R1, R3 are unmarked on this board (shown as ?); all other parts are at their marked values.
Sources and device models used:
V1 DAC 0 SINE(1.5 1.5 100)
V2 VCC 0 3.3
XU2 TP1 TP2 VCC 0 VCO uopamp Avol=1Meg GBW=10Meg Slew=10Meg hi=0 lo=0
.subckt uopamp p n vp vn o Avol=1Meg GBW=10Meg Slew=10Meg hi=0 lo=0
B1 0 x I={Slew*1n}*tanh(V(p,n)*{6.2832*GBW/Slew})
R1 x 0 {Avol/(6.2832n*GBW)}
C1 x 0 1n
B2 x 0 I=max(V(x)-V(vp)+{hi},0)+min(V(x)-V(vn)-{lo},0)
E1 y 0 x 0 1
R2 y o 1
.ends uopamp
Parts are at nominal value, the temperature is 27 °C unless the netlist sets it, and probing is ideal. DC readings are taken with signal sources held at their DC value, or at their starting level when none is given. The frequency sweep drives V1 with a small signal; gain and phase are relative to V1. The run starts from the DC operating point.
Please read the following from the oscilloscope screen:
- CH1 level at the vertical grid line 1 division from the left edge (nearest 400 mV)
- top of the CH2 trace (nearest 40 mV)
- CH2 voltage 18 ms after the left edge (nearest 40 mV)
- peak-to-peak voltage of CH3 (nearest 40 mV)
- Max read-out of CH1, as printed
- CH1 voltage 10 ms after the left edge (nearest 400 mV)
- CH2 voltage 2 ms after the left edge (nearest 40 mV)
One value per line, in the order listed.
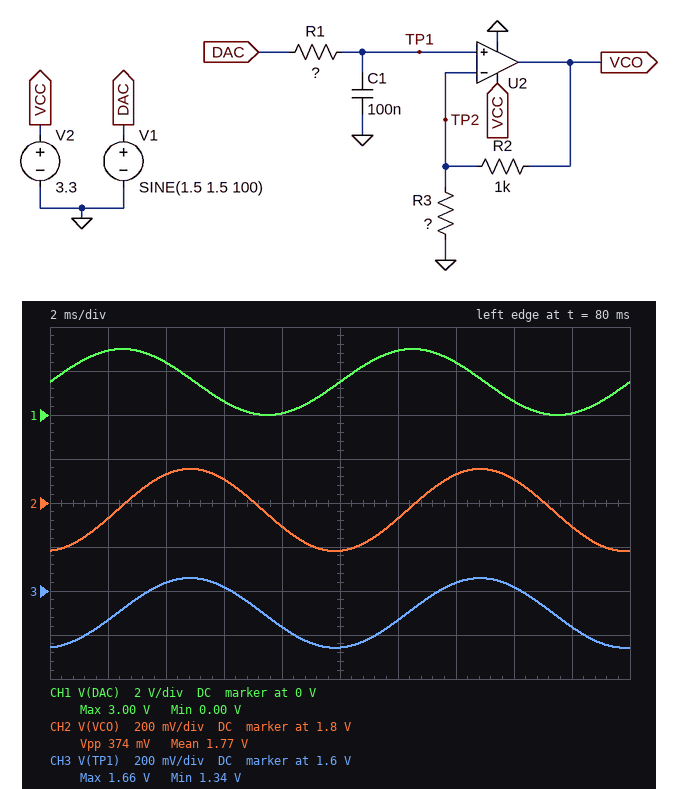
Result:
2.8 V
1.96 V
1.68 V
320 mV
3.00 V
1.6 V
1.72 V
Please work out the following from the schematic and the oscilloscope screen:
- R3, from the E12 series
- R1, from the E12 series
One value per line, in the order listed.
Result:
5.6 kΩ
150 kΩ
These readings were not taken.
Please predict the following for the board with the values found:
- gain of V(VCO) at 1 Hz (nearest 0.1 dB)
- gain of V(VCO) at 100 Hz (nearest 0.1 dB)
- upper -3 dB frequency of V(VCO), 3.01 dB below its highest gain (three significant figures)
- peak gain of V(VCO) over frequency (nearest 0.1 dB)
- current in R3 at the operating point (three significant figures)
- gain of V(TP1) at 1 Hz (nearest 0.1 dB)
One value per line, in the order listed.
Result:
1.4 dB
-18.1 dB
10.6 Hz
1.4 dB
268 µA
0 dB
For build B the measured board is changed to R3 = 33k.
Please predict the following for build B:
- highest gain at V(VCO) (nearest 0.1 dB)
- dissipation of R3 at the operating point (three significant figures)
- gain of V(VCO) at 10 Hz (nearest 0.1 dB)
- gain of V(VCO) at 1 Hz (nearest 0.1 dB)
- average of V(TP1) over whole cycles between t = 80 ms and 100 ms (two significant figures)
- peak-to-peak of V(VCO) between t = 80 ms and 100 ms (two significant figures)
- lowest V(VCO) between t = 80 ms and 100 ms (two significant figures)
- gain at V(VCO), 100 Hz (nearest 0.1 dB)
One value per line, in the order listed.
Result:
0.3 dB
68.2 µW
-2.5 dB
0.2 dB
1.5 V
330 mV
1.4 V
-19.3 dB
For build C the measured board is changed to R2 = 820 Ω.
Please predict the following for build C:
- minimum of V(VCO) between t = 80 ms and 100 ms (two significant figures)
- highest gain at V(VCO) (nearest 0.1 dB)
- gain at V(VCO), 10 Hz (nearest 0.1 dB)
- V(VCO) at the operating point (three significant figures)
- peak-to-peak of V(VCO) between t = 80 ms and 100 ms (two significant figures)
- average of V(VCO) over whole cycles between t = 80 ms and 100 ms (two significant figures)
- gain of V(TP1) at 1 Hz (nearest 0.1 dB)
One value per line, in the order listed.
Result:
1.5 V
1.2 dB
-1.6 dB
1.72 V
360 mV
1.7 V
0 dB
